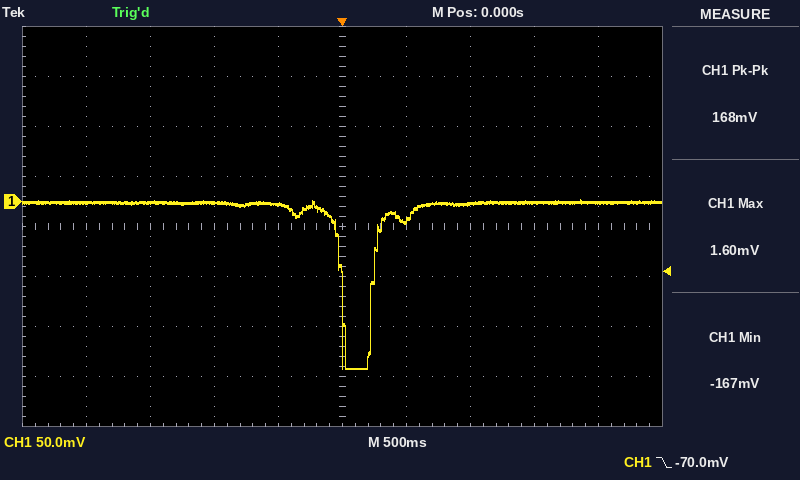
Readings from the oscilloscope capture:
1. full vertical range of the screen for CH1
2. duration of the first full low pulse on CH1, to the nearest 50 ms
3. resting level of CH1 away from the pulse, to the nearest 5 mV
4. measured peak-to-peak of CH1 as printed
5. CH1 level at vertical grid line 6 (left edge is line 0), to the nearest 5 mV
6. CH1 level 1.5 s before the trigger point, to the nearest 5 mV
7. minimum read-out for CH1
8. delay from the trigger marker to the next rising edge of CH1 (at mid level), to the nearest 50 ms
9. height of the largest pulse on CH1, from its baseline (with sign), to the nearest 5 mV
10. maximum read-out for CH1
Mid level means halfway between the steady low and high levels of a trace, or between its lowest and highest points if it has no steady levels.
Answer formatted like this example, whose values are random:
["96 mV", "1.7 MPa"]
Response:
["400 mV", "250 ms", "0 mV", "168 mV", "-20 mV", "0 mV", "-167 mV", "250 ms", "-165 mV", "1.60 mV"]
